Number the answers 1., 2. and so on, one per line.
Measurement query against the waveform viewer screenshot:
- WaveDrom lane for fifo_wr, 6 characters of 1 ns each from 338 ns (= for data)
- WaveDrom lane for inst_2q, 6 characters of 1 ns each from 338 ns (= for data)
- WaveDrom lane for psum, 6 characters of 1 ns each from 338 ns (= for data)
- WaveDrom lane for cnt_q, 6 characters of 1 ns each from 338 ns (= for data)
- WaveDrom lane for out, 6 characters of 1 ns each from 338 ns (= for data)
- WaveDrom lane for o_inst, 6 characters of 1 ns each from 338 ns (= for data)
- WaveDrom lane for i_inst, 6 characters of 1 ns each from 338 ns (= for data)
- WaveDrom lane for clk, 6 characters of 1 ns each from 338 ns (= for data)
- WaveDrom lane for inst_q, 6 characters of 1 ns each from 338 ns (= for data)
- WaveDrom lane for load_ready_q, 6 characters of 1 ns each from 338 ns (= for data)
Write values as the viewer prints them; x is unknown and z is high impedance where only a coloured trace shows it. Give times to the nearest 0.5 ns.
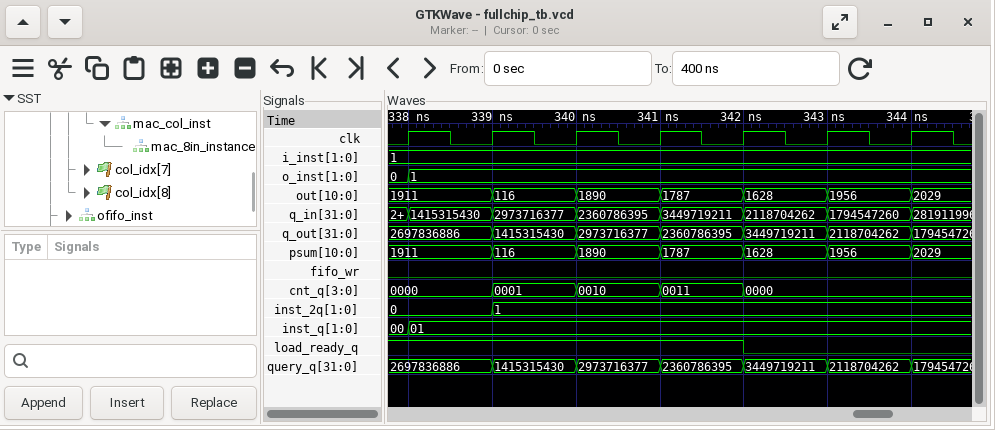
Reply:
1. {name: 'fifo_wr', wave: '0.....'}
2. {name: 'inst_2q', wave: '==....', data: '0 1'}
3. {name: 'psum', wave: '======', data: '1911 116 1890 1787 1628 1956'}
4. {name: 'cnt_q', wave: '=====.', data: '0000 0001 0010 0011 0000'}
5. {name: 'out', wave: '======', data: '1911 116 1890 1787 1628 1956'}
6. {name: 'o_inst', wave: '=.....', data: '1'}
7. {name: 'i_inst', wave: '=.....', data: '1'}
8. {name: 'clk', wave: 'p.....'}
9. {name: 'inst_q', wave: '=.....', data: '01'}
10. {name: 'load_ready_q', wave: '1...0.'}
